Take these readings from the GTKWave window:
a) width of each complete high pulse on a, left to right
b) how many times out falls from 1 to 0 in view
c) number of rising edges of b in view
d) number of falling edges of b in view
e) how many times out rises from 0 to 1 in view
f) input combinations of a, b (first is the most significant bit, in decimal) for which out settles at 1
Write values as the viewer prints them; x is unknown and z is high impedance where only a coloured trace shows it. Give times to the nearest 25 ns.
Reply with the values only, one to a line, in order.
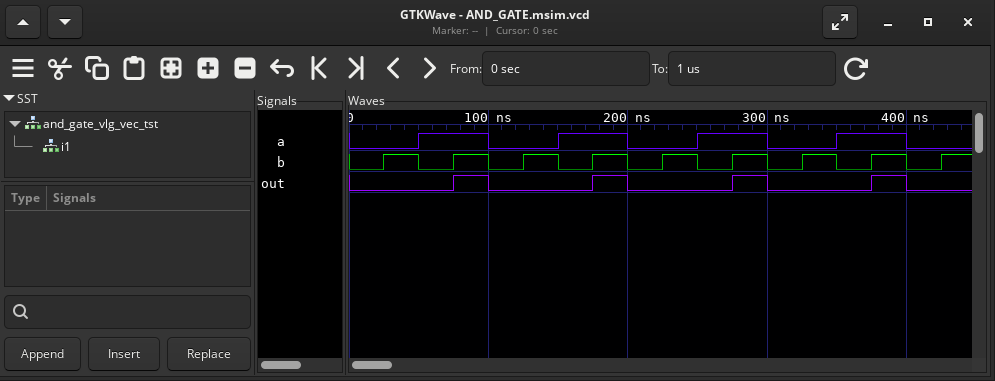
50 ns, 50 ns, 50 ns, 50 ns
4
9
8
4
3
